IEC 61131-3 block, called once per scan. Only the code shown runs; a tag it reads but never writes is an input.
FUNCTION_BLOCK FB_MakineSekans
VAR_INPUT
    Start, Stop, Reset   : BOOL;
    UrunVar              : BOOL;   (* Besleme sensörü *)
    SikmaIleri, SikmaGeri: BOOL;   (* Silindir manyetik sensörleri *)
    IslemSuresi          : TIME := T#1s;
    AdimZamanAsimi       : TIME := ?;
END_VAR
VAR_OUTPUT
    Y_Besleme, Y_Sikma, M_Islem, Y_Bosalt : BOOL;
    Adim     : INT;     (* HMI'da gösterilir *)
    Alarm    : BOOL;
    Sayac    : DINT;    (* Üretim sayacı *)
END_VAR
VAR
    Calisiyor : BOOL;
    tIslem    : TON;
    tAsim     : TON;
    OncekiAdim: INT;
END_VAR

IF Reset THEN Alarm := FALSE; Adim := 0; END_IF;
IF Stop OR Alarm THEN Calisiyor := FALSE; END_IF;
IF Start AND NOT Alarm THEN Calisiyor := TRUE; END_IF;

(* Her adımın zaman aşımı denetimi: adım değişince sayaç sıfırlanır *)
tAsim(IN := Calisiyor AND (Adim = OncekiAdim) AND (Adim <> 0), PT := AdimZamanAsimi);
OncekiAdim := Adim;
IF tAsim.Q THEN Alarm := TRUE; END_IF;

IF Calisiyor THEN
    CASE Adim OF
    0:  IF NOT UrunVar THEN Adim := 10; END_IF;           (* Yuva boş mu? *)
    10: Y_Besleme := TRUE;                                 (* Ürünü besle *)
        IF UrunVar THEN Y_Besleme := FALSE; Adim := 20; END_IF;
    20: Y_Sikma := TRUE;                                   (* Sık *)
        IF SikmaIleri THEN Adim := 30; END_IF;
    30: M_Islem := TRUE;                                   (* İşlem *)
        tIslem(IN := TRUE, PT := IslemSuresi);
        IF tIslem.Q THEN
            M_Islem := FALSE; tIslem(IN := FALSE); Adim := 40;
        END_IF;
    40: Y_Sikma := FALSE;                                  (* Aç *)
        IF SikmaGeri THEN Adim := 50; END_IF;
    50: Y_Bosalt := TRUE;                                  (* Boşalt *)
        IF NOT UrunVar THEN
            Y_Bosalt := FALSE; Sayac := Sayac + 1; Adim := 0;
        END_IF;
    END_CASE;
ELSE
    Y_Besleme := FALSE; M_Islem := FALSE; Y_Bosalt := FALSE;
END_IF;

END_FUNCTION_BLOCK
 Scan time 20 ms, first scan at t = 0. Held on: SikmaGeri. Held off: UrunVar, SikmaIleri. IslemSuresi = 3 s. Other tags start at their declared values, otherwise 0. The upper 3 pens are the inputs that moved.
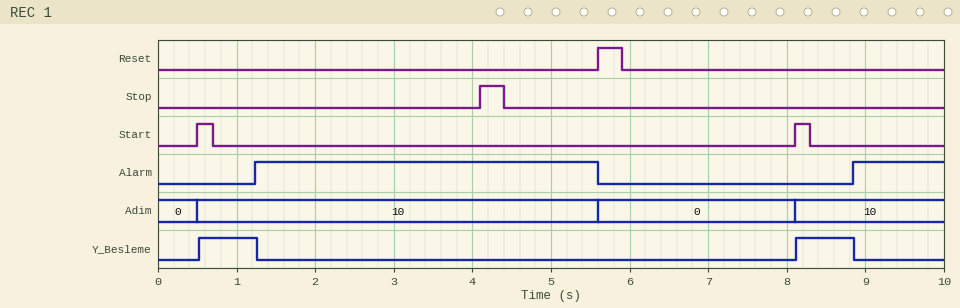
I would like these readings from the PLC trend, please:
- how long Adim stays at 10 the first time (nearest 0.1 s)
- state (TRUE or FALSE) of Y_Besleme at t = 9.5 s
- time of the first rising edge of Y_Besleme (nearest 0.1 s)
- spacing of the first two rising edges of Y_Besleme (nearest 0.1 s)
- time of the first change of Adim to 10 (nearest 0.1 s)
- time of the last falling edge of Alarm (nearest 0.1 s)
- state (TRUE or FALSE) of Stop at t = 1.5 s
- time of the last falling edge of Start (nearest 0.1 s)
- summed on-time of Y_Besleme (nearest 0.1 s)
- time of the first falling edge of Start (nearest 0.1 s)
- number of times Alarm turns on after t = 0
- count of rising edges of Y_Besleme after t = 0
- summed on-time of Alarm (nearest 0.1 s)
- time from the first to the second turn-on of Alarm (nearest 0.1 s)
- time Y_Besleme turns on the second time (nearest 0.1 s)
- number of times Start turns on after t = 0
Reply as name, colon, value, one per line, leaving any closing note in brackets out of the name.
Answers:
how long Adim stays at 10 the first time: 5.1 s
state (TRUE or FALSE) of Y_Besleme at t = 9.5 s: FALSE
time of the first rising edge of Y_Besleme: 0.5 s
spacing of the first two rising edges of Y_Besleme: 7.6 s
time of the first change of Adim to 10: 0.5 s
time of the last falling edge of Alarm: 5.6 s
state (TRUE or FALSE) of Stop at t = 1.5 s: FALSE
time of the last falling edge of Start: 8.3 s
summed on-time of Y_Besleme: 1.5 s
time of the first falling edge of Start: 0.7 s
number of times Alarm turns on after t = 0: 2
count of rising edges of Y_Besleme after t = 0: 2
summed on-time of Alarm: 5.5 s
time from the first to the second turn-on of Alarm: 7.6 s
time Y_Besleme turns on the second time: 8.1 s
number of times Start turns on after t = 0: 2
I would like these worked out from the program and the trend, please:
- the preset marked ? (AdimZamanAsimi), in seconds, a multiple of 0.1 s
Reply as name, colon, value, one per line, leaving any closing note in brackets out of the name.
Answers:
the preset marked ? (AdimZamanAsimi), in seconds, a multiple of 0.1 s: 0.7 s
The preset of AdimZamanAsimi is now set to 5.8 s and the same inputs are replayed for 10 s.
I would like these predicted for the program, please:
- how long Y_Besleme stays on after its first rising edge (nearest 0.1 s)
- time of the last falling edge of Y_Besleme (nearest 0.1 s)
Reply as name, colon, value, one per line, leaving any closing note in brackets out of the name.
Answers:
how long Y_Besleme stays on after its first rising edge: 3.6 s
time of the last falling edge of Y_Besleme: 4.1 s
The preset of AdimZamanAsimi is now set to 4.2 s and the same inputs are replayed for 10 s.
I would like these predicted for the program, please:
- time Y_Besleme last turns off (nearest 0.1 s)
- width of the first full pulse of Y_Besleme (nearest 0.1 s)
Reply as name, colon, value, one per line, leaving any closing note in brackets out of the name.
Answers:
time Y_Besleme last turns off: 4.1 s
width of the first full pulse of Y_Besleme: 3.6 s
